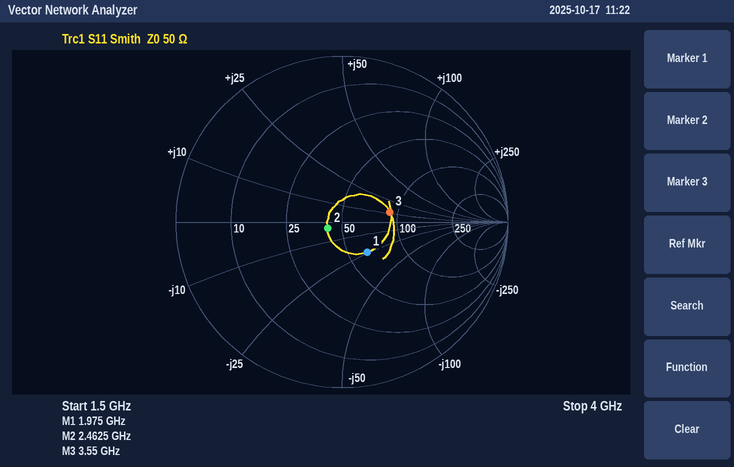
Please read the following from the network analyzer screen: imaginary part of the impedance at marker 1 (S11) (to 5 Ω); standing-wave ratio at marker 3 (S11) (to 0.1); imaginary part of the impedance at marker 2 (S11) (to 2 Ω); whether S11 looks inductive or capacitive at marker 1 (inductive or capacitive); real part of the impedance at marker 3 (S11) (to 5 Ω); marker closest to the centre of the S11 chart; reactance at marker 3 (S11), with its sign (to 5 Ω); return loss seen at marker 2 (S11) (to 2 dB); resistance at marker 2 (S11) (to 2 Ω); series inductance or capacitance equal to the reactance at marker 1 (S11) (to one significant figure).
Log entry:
-25 Ω
1.8
-4 Ω
capacitive
90 Ω
marker 2
+10 Ω
20 dB
42 Ω
3 pF
